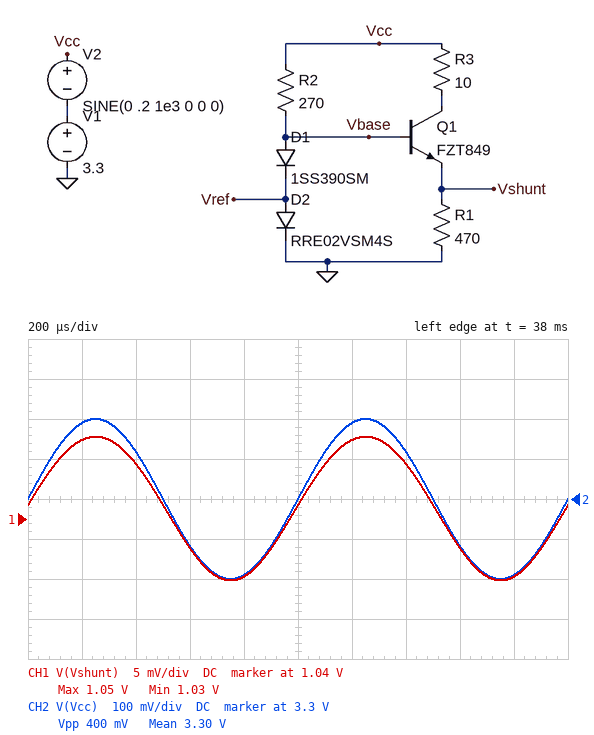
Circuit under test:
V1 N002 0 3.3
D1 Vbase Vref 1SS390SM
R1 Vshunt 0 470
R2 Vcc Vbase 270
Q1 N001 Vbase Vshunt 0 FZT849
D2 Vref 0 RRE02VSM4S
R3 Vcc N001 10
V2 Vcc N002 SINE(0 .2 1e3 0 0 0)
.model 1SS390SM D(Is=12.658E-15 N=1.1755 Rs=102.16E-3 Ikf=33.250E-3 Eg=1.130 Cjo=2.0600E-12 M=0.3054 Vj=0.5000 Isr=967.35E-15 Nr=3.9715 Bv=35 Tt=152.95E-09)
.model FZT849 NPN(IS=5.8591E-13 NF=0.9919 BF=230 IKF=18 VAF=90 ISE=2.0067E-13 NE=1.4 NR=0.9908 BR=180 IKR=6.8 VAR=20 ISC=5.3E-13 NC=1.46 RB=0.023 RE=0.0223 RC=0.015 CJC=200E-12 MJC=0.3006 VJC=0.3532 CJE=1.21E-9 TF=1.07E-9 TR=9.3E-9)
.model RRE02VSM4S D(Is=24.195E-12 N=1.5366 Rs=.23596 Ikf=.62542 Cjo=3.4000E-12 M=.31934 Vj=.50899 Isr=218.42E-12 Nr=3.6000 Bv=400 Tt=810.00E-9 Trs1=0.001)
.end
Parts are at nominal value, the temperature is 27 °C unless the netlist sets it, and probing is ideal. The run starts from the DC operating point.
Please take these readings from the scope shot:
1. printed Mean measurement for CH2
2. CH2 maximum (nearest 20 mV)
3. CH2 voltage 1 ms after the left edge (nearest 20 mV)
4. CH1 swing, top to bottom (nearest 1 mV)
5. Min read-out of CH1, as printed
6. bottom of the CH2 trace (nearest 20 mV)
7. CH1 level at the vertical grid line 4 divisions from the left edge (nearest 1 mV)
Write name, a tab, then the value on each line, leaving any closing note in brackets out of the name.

printed Mean measurement for CH2	3.30 V
CH2 maximum	3.50 V
CH2 voltage 1 ms after the left edge	3.30 V
CH1 swing, top to bottom	18 mV
Min read-out of CH1, as printed	1.03 V
bottom of the CH2 trace	3.10 V
CH1 level at the vertical grid line 4 divisions from the left edge	1.033 V
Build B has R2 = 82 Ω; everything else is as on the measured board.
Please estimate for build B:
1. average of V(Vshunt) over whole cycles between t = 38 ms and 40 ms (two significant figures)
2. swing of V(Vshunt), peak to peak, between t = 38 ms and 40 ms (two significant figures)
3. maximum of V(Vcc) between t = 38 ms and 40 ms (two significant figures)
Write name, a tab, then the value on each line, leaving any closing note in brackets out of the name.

average of V(Vshunt) over whole cycles between t = 38 ms and 40 ms	1.1 V
swing of V(Vshunt), peak to peak, between t = 38 ms and 40 ms	21 mV
maximum of V(Vcc) between t = 38 ms and 40 ms	3.5 V
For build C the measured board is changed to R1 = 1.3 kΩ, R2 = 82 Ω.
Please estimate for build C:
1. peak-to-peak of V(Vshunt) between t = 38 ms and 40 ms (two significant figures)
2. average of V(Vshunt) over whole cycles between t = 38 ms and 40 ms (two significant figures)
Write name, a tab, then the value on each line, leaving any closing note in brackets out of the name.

peak-to-peak of V(Vshunt) between t = 38 ms and 40 ms	21 mV
average of V(Vshunt) over whole cycles between t = 38 ms and 40 ms	1.2 V
